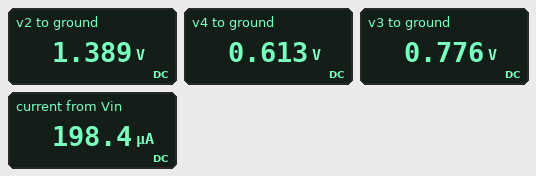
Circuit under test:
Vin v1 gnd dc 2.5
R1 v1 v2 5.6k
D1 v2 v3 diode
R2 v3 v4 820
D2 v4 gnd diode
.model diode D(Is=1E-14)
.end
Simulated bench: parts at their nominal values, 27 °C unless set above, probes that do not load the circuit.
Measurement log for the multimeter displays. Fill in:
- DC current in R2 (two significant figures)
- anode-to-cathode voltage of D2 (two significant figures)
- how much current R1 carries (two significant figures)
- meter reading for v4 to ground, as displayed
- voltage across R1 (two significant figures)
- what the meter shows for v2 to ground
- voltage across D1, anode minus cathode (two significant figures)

200 µA
610 mV
200 µA
0.613 V
1.1 V
1.389 V
610 mV
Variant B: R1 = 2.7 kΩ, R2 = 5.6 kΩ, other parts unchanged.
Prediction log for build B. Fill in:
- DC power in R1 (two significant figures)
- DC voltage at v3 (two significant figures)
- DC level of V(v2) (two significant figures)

65 µW
1.5 V
2.1 V
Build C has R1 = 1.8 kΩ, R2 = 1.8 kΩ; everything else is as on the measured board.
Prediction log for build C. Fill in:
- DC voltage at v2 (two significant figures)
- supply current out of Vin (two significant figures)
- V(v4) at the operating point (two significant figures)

1.9 V
350 µA
630 mV
